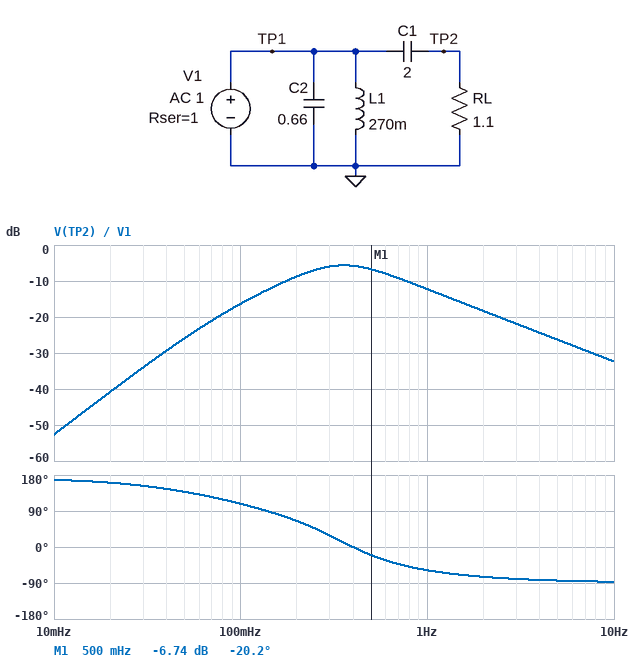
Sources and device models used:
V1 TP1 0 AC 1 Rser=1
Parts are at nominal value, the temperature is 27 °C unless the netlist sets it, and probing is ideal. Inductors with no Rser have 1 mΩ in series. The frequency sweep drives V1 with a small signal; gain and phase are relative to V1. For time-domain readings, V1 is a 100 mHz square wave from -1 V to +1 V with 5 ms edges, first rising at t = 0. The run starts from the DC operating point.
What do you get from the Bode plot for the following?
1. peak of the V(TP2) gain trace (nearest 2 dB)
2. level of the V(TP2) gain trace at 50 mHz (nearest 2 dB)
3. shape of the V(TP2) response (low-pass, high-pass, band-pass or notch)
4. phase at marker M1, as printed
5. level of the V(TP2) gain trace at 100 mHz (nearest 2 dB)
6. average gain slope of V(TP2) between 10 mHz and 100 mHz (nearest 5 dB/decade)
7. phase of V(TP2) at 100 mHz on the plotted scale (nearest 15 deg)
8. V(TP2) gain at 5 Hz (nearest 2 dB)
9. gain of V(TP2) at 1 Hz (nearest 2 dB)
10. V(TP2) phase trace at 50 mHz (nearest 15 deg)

-6 dB
-26 dB
band-pass
-20.2 deg
-16 dB
35 dB/decade
105 deg
-26 dB
-12 dB
135 deg
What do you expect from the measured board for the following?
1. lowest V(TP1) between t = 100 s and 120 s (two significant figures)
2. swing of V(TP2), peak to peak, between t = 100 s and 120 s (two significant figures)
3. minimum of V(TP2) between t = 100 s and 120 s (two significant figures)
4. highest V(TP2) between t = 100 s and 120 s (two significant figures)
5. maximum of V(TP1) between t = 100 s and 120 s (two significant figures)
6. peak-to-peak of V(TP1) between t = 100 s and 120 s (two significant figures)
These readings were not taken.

-650 mV
1.2 V
-590 mV
590 mV
650 mV
1.3 V
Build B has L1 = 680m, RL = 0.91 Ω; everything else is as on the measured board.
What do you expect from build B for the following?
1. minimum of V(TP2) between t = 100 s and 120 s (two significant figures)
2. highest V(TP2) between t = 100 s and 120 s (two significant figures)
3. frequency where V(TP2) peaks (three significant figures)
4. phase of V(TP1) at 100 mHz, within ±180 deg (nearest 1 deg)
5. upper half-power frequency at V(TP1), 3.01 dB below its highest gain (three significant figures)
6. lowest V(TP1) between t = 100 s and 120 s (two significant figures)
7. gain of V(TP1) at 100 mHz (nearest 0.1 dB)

-750 mV
750 mV
195 mHz
40 deg
475 mHz
-820 mV
-6.6 dB
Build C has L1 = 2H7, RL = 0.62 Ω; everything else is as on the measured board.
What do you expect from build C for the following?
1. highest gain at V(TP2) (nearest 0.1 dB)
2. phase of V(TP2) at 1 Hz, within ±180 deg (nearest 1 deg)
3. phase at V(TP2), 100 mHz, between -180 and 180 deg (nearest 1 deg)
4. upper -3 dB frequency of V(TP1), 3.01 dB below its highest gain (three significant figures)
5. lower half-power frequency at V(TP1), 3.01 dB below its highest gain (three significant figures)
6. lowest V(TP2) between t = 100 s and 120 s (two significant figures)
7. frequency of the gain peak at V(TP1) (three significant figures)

-8.9 dB
-52 deg
31 deg
108 mHz
30.5 mHz
-580 mV
53.9 mHz
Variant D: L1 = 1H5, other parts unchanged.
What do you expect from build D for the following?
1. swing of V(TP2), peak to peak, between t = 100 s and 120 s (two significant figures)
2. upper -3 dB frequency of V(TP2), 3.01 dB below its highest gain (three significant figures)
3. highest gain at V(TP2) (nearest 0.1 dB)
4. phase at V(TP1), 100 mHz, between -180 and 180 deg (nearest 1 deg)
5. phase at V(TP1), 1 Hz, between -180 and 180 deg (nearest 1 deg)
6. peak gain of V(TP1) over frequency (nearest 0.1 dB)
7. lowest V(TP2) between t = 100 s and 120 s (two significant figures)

1.7 V
492 mHz
-5.8 dB
8 deg
-65 deg
-4.0 dB
-870 mV
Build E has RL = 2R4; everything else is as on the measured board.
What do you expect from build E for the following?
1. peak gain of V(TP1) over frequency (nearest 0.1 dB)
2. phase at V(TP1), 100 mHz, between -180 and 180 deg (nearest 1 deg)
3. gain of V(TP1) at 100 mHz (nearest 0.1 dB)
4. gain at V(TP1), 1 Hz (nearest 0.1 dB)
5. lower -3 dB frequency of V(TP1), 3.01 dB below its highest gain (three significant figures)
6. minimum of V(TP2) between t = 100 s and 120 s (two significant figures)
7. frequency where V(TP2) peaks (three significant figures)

-3.0 dB
75 deg
-14.9 dB
-11.7 dB
239 mHz
-720 mV
373 mHz
